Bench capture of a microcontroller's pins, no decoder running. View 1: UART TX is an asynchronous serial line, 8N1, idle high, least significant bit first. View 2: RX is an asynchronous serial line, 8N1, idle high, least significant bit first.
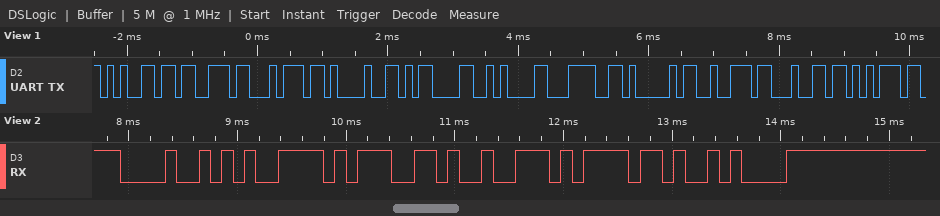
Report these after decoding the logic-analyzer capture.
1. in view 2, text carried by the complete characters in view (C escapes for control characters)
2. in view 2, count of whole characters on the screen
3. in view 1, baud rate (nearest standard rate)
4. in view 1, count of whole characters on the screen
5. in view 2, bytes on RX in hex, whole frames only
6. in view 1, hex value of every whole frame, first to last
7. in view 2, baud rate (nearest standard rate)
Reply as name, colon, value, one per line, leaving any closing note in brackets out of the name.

in view 2, text carried by the complete characters in view: "Hygro\n"
in view 2, count of whole characters on the screen: 6
in view 1, baud rate: 9600 baud
in view 1, count of whole characters on the screen: 11
in view 2, bytes on RX in hex, whole frames only: 0x48 0x79 0x67 0x72 0x6F 0x0A
in view 1, hex value of every whole frame, first to last: 65 73 74 21 0D 0A 3C 41 72 64 75
in view 2, baud rate: 9600 baud
